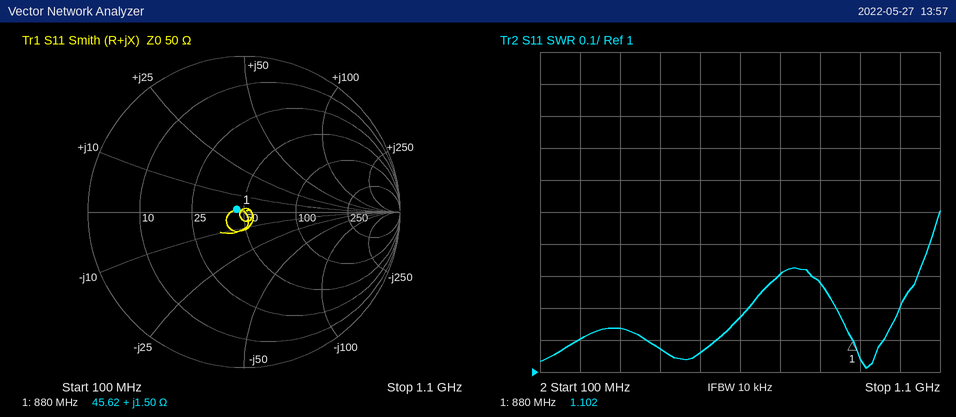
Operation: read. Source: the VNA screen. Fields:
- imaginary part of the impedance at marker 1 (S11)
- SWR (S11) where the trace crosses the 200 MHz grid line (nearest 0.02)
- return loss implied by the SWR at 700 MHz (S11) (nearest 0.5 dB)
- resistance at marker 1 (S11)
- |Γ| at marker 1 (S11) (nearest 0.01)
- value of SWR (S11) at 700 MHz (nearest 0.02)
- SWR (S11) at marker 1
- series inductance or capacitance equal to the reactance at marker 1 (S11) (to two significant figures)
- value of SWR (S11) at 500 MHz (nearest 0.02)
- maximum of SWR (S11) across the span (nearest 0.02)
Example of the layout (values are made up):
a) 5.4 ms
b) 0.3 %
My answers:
a) +1.50 Ω
b) 1.10
c) 17.5 dB
d) 45.62 Ω
e) 0.05
f) 1.30
g) 1.102
h) 270 pH
i) 1.06
j) 1.50
